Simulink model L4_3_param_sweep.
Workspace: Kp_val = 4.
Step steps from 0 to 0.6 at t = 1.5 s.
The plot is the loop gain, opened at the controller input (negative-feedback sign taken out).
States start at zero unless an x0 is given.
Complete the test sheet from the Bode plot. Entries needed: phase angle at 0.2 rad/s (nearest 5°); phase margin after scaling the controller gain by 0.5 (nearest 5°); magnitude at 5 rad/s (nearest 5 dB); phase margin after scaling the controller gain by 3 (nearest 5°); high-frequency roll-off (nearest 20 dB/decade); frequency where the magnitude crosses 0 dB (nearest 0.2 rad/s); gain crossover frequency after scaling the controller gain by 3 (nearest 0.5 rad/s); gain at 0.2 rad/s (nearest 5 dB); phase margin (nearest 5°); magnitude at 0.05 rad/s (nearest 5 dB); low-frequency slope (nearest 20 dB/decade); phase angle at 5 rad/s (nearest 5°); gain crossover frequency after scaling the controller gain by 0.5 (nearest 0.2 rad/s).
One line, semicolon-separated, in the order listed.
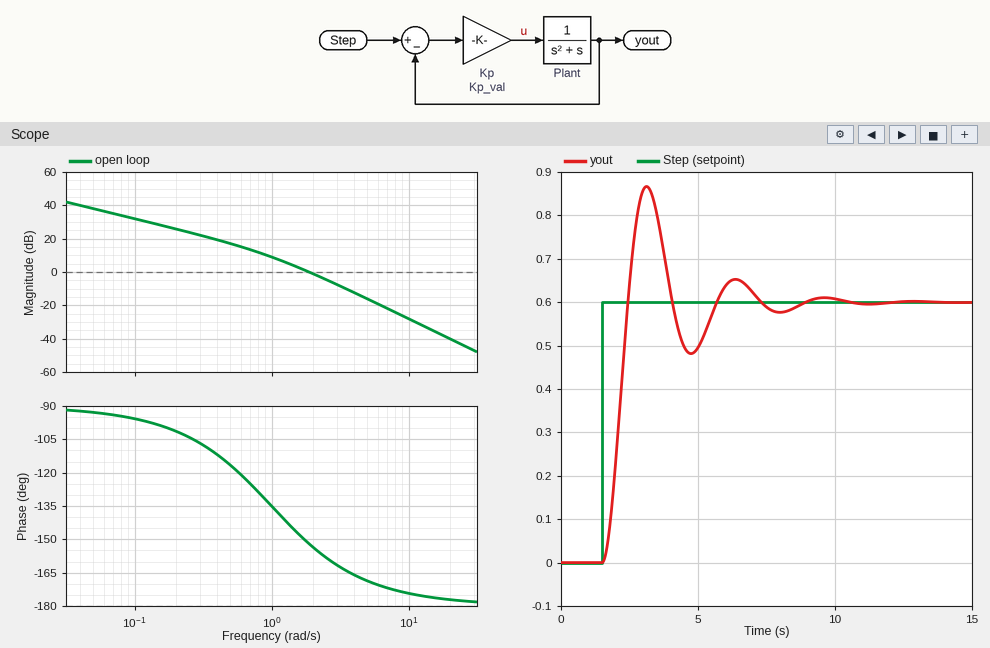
-100°; 40°; -15 dB; 15°; -40 dB/decade; 1.8 rad/s; 3.5 rad/s; 25 dB; 30°; 40 dB; -20 dB/decade; -170°; 1.2 rad/s
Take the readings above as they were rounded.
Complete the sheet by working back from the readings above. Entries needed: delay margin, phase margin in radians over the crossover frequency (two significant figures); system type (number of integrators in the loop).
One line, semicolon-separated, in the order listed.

0.29 s; 1
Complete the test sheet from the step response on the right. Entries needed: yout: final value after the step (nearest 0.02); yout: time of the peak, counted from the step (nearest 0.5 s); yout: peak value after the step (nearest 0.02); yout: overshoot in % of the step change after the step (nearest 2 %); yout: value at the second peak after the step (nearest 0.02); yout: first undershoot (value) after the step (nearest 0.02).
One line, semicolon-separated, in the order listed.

0.60; 1.5 s; 0.86; 44 %; 0.66; 0.48
